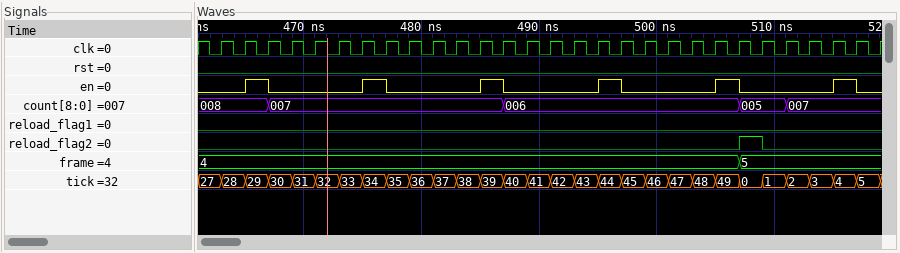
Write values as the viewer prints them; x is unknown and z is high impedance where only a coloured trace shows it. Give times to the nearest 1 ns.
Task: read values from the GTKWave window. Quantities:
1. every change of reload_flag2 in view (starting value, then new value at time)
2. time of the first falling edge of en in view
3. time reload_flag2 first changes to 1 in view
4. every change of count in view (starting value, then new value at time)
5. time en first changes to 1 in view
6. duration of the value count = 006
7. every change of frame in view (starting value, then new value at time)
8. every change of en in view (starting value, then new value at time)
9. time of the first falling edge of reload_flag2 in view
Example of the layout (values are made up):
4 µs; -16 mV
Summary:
0, 1 at 507 ns, 0 at 509 ns; 467 ns; 507 ns; 008, 007 at 467 ns, 006 at 487 ns, 005 at 507 ns, 007 at 511 ns; 465 ns; 20 ns; 4, 5 at 507 ns; 0, 1 at 465 ns, 0 at 467 ns, 1 at 475 ns, 0 at 477 ns, 1 at 485 ns, 0 at 487 ns, 1 at 495 ns, 0 at 497 ns, 1 at 505 ns, 0 at 507 ns, 1 at 515 ns, 0 at 517 ns; 509 ns
